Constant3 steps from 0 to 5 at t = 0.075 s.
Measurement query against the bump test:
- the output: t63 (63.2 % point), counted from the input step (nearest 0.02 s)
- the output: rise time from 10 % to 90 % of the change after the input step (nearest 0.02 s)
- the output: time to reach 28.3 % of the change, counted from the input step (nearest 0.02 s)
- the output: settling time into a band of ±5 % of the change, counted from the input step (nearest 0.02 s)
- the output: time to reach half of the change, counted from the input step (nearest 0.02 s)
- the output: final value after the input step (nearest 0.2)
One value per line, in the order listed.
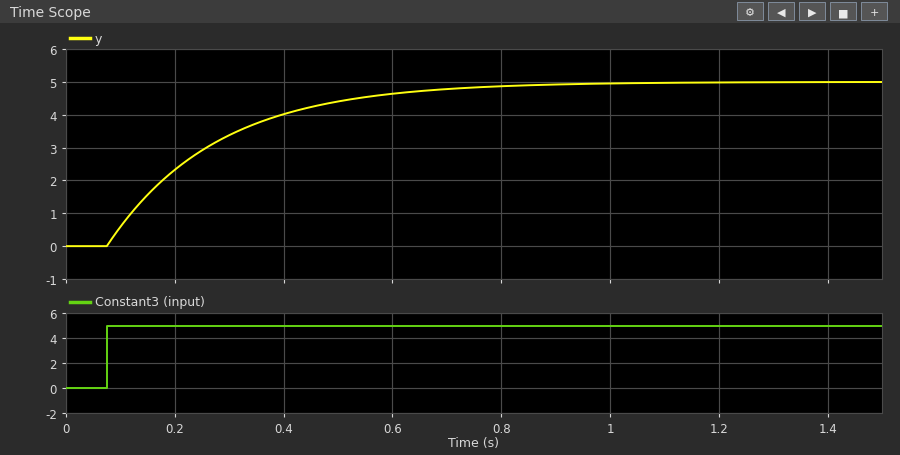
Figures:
0.20 s
0.44 s
0.06 s
0.60 s
0.14 s
5.0
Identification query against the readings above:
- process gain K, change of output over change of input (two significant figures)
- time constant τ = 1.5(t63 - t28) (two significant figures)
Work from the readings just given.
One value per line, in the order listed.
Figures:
1.0
0.21 s
